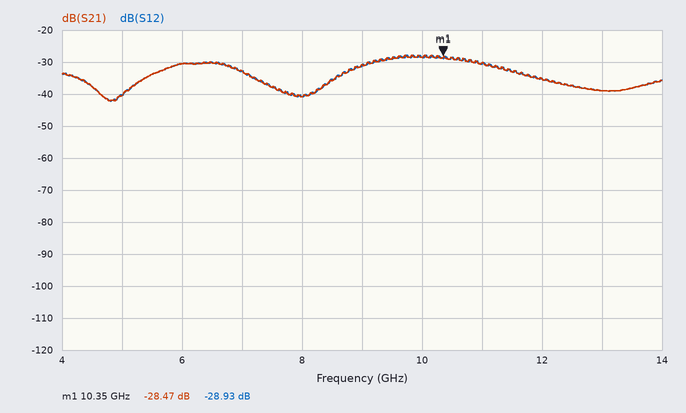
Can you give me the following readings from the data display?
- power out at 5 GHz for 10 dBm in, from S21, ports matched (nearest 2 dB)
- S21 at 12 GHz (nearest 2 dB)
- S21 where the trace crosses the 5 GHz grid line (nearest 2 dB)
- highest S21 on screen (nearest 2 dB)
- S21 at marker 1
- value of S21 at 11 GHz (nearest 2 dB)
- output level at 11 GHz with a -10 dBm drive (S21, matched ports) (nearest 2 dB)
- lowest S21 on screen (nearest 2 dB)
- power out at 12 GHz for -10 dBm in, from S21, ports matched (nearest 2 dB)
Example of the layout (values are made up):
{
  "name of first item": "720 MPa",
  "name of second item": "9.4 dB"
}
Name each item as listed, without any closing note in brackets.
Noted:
{
  "power out at 5 GHz for 10 dBm in, from S21, ports matched": "-30 dBm",
  "S21 at 12 GHz": "-36 dB",
  "S21 where the trace crosses the 5 GHz grid line": "-40 dB",
  "highest S21 on screen": "-28 dB",
  "S21 at marker 1": "-28.47 dB",
  "value of S21 at 11 GHz": "-30 dB",
  "output level at 11 GHz with a -10 dBm drive (S21, matched ports)": "-40 dBm",
  "lowest S21 on screen": "-42 dB",
  "power out at 12 GHz for -10 dBm in, from S21, ports matched": "-46 dBm"
}
